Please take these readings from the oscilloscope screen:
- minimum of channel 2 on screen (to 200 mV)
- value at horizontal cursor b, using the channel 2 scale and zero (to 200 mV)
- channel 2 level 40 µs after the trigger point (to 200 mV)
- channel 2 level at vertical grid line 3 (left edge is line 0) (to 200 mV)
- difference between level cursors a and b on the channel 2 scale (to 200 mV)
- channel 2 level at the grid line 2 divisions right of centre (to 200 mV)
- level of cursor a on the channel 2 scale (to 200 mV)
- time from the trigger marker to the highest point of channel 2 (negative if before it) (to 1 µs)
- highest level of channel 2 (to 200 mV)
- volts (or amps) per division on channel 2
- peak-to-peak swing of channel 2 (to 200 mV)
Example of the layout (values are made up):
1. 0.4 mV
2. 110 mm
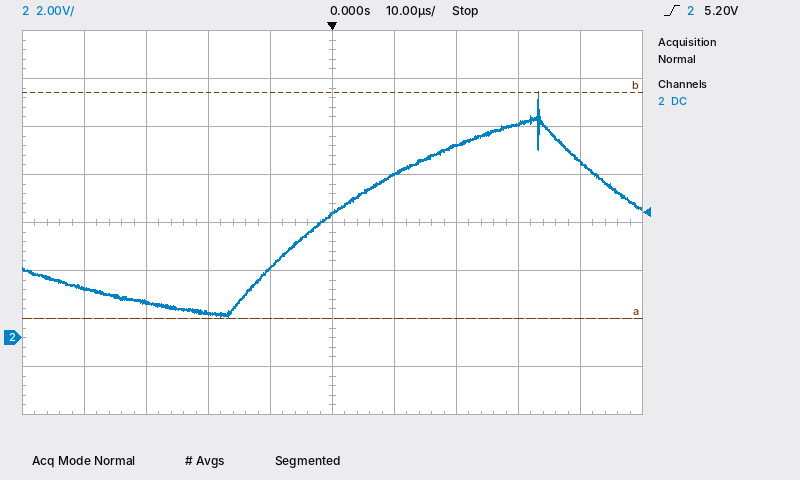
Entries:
1. 800 mV
2. 10.2 V
3. 7.4 V
4. 1.0 V
5. 9.4 V
6. 8.0 V
7. 800 mV
8. +33 µs
9. 10.2 V
10. 2 V
11. 9.4 V
